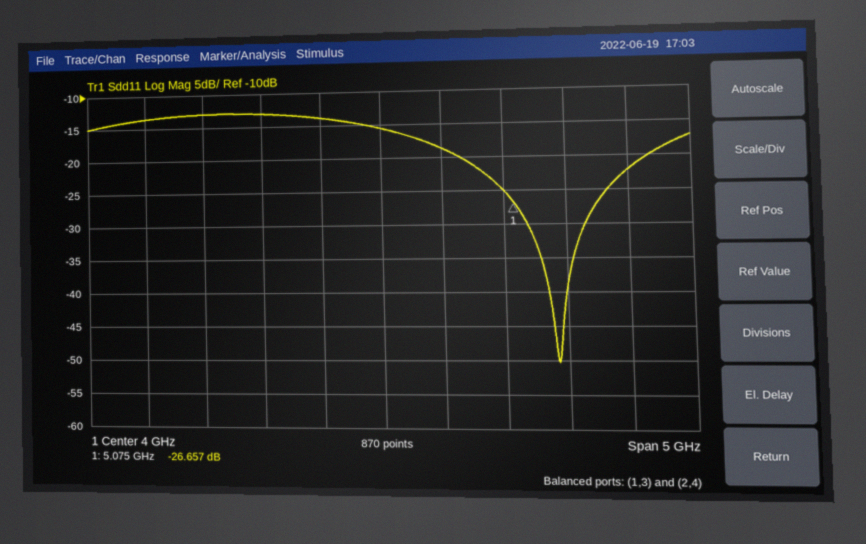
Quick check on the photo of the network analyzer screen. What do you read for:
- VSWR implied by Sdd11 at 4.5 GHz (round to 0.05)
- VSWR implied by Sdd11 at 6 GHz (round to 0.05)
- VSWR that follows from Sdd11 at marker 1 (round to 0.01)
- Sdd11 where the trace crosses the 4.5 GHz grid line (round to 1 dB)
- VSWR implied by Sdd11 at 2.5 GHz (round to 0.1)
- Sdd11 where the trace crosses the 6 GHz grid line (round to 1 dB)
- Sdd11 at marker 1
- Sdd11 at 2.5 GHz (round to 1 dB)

1.25
1.15
1.10
-19 dB
1.6
-22 dB
-26.657 dB
-13 dB
